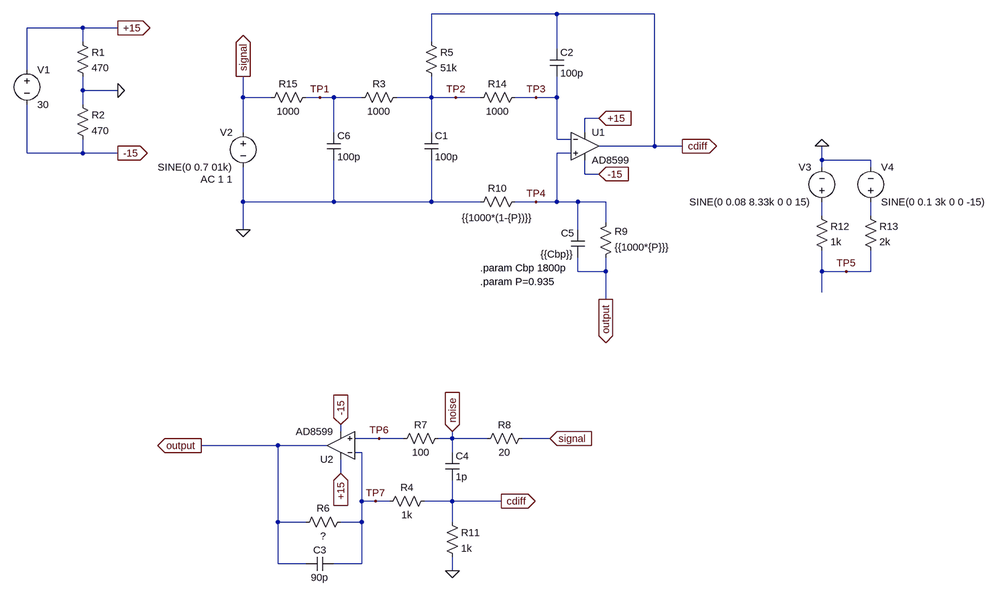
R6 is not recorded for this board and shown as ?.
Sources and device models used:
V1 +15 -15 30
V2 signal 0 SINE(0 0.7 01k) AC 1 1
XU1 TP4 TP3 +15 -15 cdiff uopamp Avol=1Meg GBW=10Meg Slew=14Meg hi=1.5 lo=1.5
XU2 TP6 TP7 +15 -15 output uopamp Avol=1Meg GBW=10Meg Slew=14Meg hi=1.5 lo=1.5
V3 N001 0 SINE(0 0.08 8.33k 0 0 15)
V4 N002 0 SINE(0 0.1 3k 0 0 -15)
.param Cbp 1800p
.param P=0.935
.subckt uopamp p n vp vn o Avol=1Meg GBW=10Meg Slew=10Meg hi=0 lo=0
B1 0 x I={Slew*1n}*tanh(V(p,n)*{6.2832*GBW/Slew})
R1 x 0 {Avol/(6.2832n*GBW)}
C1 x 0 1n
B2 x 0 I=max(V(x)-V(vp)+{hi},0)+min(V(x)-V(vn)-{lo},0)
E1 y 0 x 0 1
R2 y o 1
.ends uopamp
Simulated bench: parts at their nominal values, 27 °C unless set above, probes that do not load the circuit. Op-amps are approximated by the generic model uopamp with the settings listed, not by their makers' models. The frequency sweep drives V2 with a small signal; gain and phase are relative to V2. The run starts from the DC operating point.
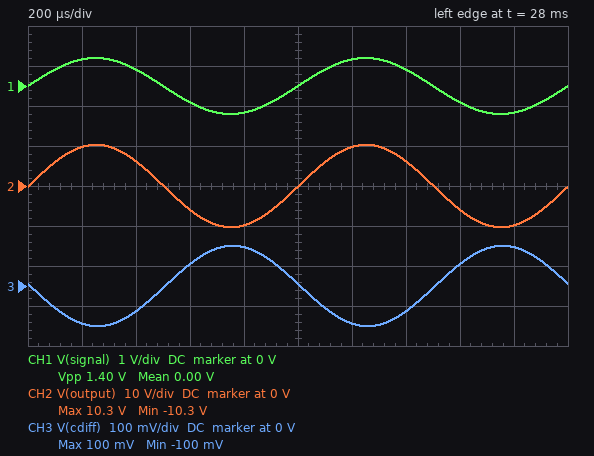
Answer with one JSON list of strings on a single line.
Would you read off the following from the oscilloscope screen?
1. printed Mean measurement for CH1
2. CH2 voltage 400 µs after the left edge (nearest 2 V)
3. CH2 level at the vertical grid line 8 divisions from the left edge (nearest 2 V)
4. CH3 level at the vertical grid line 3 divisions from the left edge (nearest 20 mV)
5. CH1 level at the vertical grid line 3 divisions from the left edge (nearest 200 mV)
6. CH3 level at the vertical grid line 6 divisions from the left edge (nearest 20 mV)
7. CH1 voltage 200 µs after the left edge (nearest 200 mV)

["0.00 V", "6 V", "-6 V", "60 mV", "-400 mV", "-100 mV", "600 mV"]
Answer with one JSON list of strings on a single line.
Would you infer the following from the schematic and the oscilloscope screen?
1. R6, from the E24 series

["12 kΩ"]
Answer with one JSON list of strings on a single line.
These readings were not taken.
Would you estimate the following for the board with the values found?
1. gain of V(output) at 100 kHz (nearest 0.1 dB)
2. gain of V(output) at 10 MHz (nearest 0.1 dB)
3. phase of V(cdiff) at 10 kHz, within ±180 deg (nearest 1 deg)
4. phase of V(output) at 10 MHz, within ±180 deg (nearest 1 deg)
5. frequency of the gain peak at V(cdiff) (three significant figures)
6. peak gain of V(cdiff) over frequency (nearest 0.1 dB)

["19.1 dB", "-3.0 dB", "152 deg", "-50 deg", "2.51 MHz", "0.6 dB"]
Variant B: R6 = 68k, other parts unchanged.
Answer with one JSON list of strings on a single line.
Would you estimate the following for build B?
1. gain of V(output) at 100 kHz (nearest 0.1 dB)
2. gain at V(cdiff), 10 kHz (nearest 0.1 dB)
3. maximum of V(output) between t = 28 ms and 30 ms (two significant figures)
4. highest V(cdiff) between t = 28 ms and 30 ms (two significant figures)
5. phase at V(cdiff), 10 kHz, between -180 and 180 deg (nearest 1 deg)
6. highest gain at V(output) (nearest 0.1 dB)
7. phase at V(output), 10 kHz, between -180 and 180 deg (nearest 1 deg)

["20.1 dB", "-2.1 dB", "11 V", "550 mV", "-5 deg", "23.7 dB", "-7 deg"]
